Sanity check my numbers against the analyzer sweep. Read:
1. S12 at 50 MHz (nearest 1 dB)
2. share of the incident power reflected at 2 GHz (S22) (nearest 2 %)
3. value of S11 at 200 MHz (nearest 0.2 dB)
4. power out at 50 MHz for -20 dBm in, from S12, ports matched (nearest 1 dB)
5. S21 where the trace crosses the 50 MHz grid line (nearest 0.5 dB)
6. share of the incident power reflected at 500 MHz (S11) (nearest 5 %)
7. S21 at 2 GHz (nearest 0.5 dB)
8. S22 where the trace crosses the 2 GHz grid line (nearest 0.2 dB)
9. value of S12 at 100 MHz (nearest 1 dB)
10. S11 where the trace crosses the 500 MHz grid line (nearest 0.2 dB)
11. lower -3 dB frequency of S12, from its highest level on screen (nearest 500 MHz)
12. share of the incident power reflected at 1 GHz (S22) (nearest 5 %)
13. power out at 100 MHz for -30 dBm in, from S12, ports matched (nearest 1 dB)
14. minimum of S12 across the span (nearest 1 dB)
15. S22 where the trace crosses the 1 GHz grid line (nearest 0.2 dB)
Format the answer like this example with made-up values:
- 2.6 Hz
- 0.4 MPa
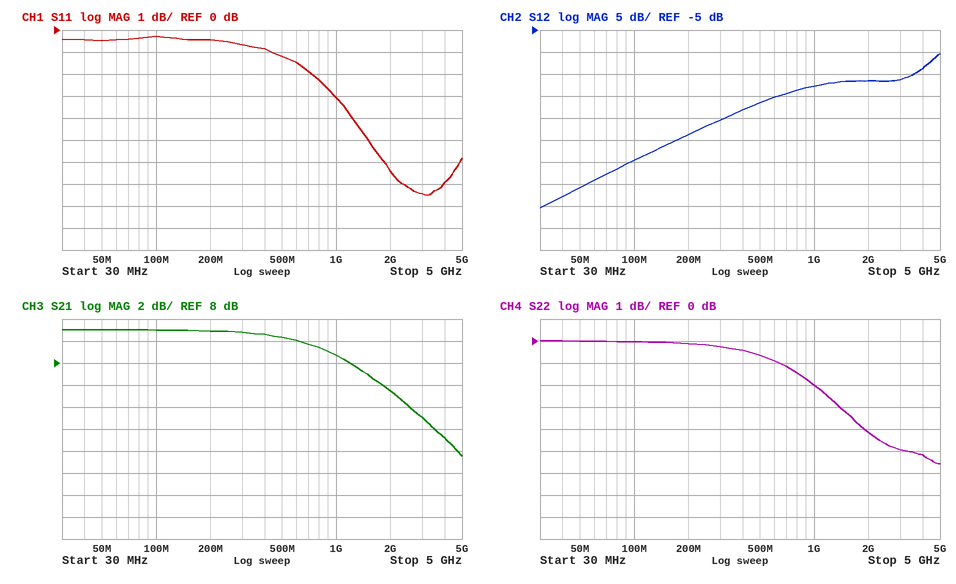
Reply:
- -41 dB
- 38 %
- -0.4 dB
- -61 dBm
- 11.0 dB
- 75 %
- 5.5 dB
- -4.2 dB
- -35 dB
- -1.2 dB
- 4.0 GHz
- 65 %
- -65 dBm
- -45 dB
- -2.0 dB
